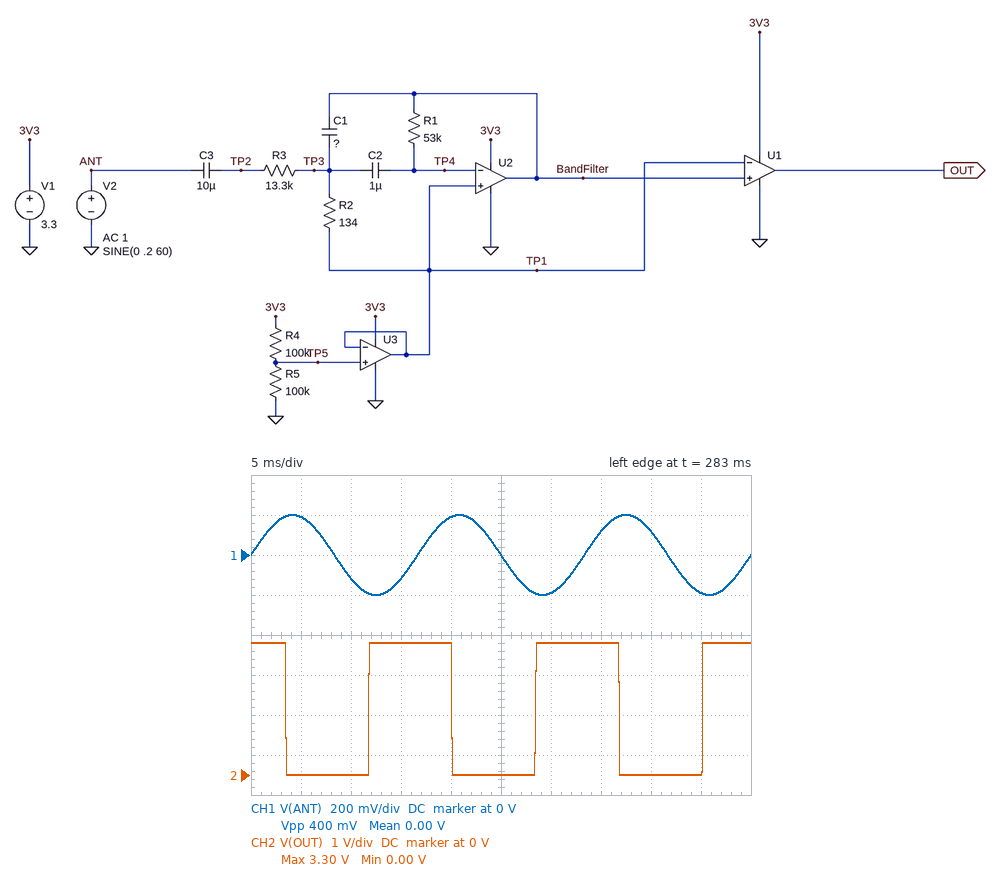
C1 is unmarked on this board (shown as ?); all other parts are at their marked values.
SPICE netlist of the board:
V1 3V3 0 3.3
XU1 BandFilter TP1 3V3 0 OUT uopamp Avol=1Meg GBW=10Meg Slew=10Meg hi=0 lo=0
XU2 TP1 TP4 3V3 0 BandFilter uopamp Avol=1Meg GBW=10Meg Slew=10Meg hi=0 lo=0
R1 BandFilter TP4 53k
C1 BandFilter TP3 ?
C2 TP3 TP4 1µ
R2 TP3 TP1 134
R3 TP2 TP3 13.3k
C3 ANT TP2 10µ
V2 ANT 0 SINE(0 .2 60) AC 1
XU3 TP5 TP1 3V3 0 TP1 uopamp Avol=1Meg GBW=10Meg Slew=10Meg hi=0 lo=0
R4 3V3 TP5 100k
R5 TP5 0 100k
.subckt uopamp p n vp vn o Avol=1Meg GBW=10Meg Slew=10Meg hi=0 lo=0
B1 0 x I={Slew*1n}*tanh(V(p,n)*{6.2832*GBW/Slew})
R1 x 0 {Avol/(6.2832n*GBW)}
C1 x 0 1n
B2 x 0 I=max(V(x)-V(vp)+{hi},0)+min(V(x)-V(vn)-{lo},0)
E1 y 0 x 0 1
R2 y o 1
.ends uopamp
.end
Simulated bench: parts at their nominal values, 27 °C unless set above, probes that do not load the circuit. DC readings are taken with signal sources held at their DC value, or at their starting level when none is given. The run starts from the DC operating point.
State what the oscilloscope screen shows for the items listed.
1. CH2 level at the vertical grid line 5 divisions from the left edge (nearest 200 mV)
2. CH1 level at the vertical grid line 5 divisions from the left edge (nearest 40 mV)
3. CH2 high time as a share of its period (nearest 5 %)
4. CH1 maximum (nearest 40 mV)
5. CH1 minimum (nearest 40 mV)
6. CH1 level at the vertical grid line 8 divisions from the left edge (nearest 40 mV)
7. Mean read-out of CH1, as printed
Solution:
0 V
0 V
50 %
200 mV
-200 mV
120 mV
0.00 V
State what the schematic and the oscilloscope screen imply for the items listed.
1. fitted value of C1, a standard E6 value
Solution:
1.5 µF
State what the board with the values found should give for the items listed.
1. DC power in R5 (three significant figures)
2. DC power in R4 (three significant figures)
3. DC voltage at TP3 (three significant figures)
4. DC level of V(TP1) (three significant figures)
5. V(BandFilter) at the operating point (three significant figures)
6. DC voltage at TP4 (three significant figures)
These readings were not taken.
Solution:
27.2 µW
27.2 µW
1.65 V
1.65 V
1.65 V
1.65 V
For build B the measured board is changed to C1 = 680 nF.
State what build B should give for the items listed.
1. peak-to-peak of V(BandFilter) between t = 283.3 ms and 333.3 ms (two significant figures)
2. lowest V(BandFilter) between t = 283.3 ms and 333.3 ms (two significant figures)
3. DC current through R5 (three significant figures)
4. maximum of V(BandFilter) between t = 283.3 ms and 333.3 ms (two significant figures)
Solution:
240 mV
1.5 V
16.5 µA
1.8 V
